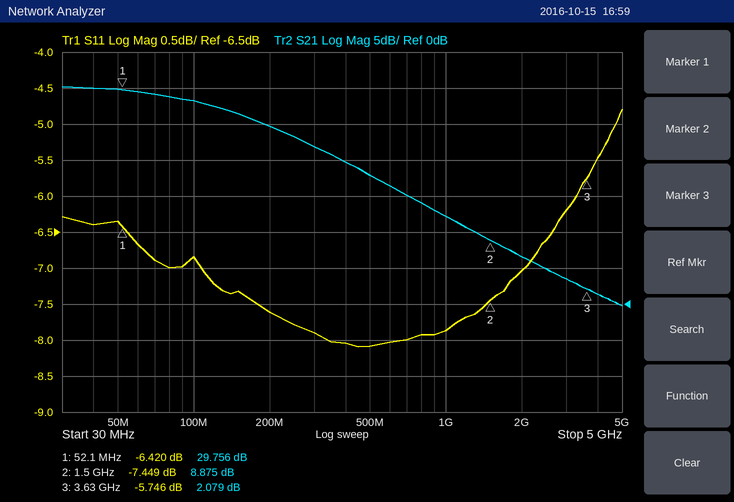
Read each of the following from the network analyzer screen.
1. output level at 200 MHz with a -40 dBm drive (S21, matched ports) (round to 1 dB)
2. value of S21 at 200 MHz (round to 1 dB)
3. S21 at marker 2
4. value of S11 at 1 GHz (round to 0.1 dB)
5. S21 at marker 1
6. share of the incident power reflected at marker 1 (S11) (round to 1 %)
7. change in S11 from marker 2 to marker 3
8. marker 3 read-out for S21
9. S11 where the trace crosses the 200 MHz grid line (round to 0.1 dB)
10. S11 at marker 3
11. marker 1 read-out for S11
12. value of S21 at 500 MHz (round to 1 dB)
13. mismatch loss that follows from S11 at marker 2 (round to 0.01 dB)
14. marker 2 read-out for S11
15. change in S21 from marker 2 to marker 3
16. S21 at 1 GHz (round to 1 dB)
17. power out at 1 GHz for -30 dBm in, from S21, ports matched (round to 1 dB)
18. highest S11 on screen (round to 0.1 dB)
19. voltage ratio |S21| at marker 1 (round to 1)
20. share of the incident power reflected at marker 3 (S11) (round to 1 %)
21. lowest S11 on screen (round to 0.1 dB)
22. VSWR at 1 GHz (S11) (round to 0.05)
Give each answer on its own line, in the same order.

-15 dBm
25 dB
8.875 dB
-7.9 dB
29.756 dB
23 %
1.703 dB
2.079 dB
-7.6 dB
-5.746 dB
-6.420 dB
18 dB
0.86 dB
-7.449 dB
-6.796 dB
12 dB
-18 dBm
-4.8 dB
31
27 %
-8.1 dB
2.35
